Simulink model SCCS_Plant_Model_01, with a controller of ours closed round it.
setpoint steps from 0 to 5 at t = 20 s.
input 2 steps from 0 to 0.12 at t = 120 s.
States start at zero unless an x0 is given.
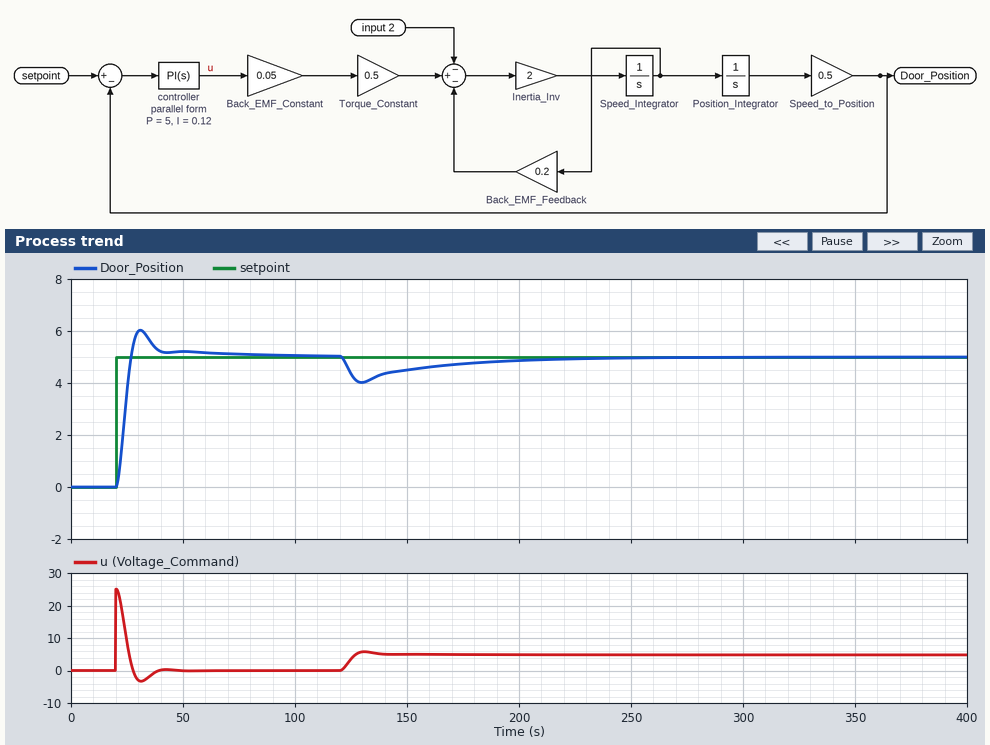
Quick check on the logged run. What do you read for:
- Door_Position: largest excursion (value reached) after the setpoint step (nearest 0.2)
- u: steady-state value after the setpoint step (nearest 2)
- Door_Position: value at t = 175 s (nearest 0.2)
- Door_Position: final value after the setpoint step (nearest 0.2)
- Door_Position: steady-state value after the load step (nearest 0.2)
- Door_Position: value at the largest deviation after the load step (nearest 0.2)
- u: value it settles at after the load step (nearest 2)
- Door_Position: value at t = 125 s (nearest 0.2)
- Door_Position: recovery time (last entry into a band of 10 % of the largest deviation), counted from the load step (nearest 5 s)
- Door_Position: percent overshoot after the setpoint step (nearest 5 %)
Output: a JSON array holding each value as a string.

["6.0", "0", "4.8", "5.0", "5.0", "4.0", "4", "4.4", "90 s", "20 %"]
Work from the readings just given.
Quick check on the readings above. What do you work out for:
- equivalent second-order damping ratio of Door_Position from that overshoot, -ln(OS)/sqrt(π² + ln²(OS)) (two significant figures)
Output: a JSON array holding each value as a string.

["0.46"]
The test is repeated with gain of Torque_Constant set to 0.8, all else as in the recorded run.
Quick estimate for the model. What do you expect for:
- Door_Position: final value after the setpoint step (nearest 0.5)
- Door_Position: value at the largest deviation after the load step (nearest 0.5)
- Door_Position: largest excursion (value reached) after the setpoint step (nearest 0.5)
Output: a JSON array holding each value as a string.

["5.0", "4.5", "6.5"]
